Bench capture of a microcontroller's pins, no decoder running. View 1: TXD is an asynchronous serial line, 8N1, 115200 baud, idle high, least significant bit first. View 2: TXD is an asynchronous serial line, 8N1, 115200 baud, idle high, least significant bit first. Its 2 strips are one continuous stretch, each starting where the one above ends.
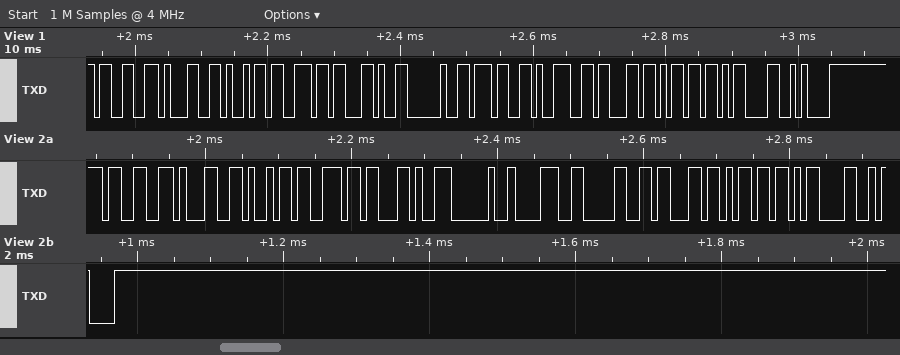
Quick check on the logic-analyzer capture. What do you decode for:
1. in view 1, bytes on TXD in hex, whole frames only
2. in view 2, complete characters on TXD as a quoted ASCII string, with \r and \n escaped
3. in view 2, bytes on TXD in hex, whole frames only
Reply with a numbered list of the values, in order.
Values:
1. 33 31 69 6E 2C 20 37 39 63 6D 0D 0A
2. "31in, 80cm\r\n"
3. 33 31 69 6E 2C 20 38 30 63 6D 0D 0A
